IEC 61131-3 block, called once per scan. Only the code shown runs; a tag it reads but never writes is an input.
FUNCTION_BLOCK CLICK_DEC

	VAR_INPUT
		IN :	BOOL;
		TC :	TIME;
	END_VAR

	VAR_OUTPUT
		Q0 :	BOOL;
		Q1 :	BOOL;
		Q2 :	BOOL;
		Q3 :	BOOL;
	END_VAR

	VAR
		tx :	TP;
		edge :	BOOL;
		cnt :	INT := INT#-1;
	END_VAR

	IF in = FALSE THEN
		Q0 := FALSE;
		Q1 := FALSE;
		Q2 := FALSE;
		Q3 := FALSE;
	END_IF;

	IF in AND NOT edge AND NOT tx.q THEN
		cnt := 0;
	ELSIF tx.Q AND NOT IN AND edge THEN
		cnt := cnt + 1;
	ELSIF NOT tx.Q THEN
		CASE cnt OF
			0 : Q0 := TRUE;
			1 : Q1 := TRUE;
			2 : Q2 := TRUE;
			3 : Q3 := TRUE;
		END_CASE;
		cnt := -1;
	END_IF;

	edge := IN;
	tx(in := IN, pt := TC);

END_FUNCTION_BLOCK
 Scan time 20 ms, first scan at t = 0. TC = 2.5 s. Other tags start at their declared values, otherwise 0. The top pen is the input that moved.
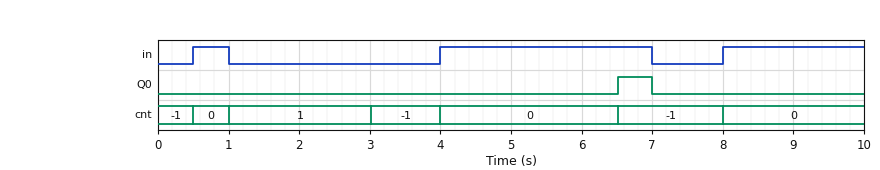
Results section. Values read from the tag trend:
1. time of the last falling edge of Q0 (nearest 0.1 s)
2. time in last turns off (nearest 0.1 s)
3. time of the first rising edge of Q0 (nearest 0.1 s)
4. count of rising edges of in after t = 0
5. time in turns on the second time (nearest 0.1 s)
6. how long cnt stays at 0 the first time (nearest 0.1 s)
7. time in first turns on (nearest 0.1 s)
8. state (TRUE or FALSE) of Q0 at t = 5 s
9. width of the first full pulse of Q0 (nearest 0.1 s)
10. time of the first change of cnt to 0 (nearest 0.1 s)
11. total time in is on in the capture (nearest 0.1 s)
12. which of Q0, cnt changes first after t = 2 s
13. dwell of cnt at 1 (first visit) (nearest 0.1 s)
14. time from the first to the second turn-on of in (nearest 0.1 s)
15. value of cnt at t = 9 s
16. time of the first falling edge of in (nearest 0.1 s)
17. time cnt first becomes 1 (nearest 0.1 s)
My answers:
7.0 s
7.0 s
6.5 s
3
4.0 s
0.5 s
0.5 s
FALSE
0.5 s
0.5 s
5.5 s
cnt
2.0 s
3.5 s
0
1.0 s
1.0 s
